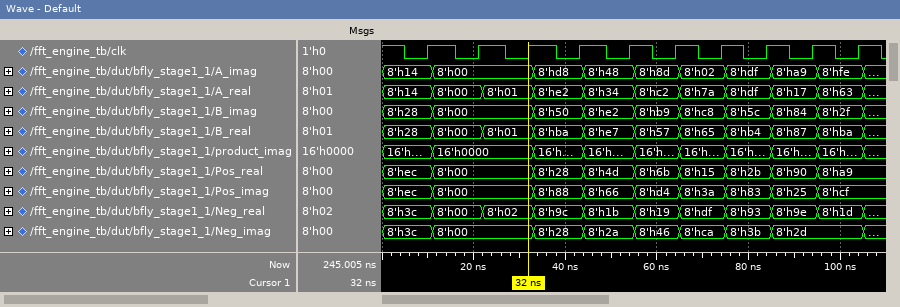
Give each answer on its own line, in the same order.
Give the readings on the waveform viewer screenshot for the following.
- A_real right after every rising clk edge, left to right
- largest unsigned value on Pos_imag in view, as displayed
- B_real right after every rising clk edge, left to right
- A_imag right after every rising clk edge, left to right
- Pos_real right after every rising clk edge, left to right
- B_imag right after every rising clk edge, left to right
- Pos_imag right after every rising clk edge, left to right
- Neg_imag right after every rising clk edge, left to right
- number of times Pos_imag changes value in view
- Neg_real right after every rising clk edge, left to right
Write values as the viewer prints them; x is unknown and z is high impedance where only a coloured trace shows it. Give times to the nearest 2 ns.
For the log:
8'h14, 8'h00, 8'h01, 8'he2, 8'h34, 8'hc2, 8'h7a, 8'hdf, 8'h17, 8'h63
8'hec
8'h28, 8'h00, 8'h01, 8'hba, 8'he7, 8'h57, 8'h65, 8'hb4, 8'h87, 8'hba
8'h14, 8'h00, 8'h00, 8'hd8, 8'h48, 8'h8d, 8'h02, 8'hdf, 8'ha9, 8'hfe
8'hec, 8'h00, 8'h00, 8'h28, 8'h4d, 8'h6b, 8'h15, 8'h2b, 8'h90, 8'ha9
8'h28, 8'h00, 8'h00, 8'h50, 8'he2, 8'hb9, 8'hc8, 8'h5c, 8'h84, 8'h2f
8'hec, 8'h00, 8'h00, 8'h88, 8'h66, 8'hd4, 8'h3a, 8'h83, 8'h25, 8'hcf
8'h3c, 8'h00, 8'h00, 8'h28, 8'h2a, 8'h46, 8'hca, 8'h3b, 8'h2d, 8'h2d
8
8'h3c, 8'h00, 8'h02, 8'h9c, 8'h1b, 8'h19, 8'hdf, 8'h93, 8'h9e, 8'h1d
